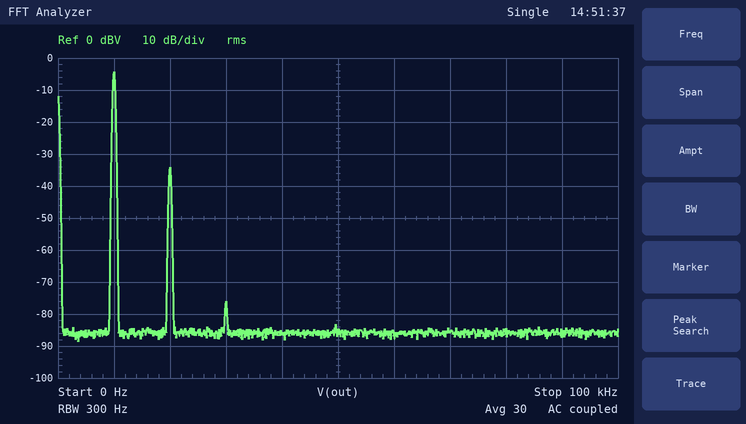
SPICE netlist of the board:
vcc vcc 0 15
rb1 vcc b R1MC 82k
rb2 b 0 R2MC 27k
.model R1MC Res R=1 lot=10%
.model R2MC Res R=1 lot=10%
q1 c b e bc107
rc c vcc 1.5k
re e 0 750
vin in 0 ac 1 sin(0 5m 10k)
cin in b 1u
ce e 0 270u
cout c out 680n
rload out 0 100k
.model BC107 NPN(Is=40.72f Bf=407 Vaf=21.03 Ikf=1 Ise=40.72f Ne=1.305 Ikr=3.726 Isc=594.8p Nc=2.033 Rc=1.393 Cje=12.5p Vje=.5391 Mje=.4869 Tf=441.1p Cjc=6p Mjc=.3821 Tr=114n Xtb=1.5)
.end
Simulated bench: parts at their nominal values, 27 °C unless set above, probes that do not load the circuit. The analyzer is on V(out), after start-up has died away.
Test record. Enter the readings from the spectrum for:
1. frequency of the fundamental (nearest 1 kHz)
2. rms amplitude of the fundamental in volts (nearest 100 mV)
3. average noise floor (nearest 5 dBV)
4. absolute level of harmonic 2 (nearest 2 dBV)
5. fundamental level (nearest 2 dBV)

10 kHz
600 mV
-85 dBV
-34 dBV
-4 dBV
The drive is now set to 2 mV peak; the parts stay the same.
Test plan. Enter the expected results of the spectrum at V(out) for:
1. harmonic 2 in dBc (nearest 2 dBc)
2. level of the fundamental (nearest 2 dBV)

-38 dBc
-12 dBV
